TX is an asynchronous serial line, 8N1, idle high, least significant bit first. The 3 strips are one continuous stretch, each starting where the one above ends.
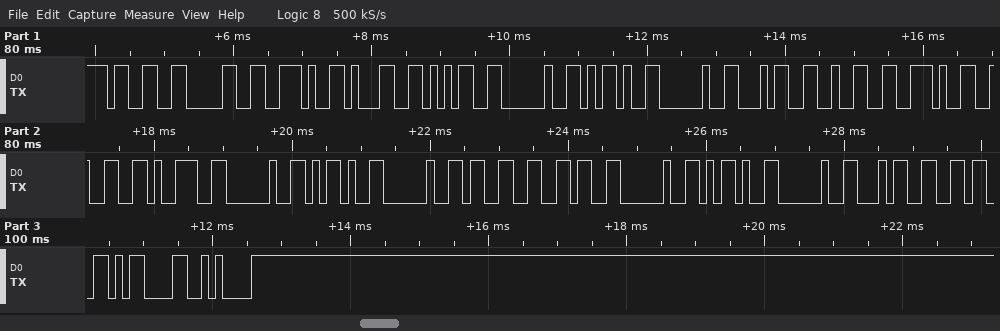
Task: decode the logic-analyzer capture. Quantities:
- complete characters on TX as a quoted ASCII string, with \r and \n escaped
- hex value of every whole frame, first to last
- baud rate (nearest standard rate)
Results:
"30.15 - 42.29 - 36 - 46\r\n"
33 30 2E 31 35 20 2D 20 34 32 2E 32 39 20 2D 20 33 36 20 2D 20 34 36 0D 0A
9600 baud
